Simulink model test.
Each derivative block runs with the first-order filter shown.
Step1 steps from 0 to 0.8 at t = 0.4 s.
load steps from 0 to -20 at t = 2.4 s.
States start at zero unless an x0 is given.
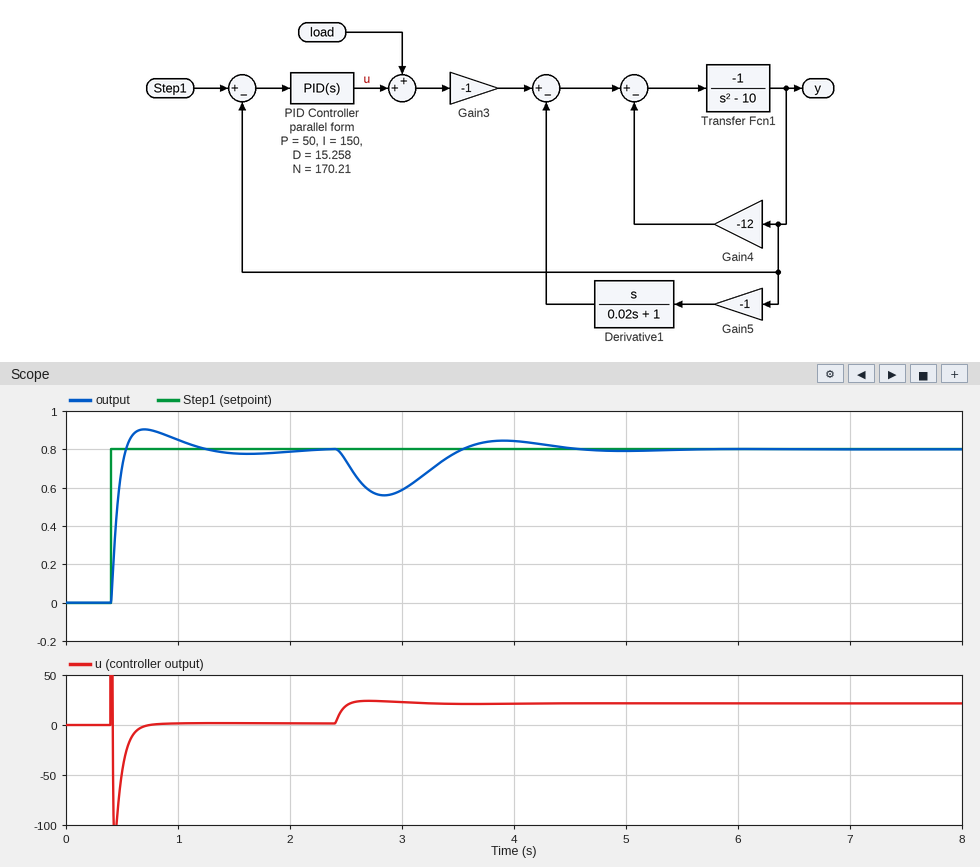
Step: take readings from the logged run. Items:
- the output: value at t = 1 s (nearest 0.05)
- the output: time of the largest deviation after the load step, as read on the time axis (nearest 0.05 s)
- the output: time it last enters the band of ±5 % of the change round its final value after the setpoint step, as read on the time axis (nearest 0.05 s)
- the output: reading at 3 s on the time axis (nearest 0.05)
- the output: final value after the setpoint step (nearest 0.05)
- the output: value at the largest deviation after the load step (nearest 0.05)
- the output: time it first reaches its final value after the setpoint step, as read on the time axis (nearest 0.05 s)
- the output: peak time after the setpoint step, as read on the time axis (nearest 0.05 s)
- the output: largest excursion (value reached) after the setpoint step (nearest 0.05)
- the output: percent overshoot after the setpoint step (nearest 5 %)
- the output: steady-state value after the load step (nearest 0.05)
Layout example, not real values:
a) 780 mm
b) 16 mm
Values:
a) 0.85
b) 2.85 s
c) 1.05 s
d) 0.60
e) 0.80
f) 0.55
g) 0.55 s
h) 0.70 s
i) 0.90
j) 15 %
k) 0.80
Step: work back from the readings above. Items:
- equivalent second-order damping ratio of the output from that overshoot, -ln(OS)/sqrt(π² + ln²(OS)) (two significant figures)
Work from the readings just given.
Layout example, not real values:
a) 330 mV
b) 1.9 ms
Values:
a) 0.52
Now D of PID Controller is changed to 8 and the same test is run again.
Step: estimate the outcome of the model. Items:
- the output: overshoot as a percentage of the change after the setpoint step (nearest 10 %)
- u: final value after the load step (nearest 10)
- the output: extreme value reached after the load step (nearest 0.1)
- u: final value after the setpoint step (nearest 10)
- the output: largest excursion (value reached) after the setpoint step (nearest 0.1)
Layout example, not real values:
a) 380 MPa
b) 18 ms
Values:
a) 30 %
b) 20
c) 0.5
d) 0
e) 1.1
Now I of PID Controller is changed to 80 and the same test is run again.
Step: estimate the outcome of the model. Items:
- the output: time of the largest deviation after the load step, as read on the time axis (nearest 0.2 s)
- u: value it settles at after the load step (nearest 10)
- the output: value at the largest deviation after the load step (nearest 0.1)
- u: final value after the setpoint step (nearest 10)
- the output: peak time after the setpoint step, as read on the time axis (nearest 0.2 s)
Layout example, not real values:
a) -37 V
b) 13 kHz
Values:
a) 3.0 s
b) 20
c) 0.5
d) 0
e) 0.6 s
